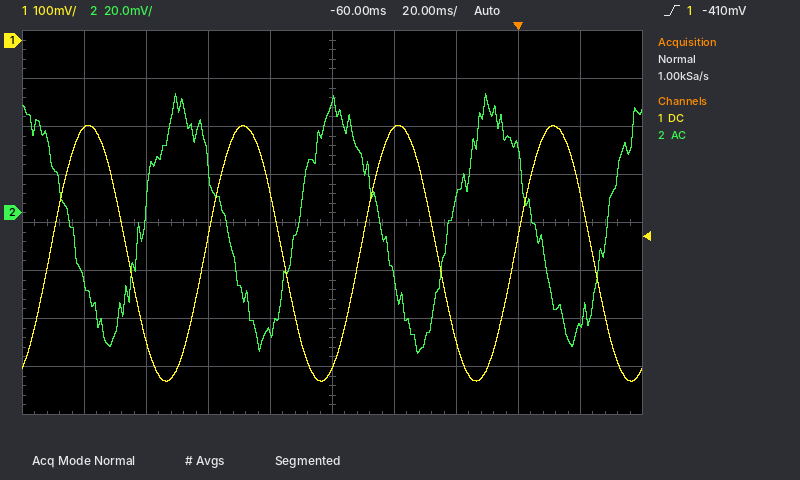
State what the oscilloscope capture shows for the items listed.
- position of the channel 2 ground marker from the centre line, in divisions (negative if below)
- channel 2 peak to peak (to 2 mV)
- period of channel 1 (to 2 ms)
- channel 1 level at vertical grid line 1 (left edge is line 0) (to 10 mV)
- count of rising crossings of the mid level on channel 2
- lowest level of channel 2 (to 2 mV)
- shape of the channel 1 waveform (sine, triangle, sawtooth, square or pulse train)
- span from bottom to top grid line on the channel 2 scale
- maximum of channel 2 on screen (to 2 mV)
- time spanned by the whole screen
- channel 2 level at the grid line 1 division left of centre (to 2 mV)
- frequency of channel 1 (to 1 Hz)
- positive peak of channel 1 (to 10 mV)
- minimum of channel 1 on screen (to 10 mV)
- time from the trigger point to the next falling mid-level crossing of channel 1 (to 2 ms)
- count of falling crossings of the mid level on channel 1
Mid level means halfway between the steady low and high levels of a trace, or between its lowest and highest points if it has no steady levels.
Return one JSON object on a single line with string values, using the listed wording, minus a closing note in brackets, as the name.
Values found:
{"position of the channel 2 ground marker from the centre line, in divisions": "+0.2 div", "channel 2 peak to peak": "108 mV", "period of channel 1": "50 ms", "channel 1 level at vertical grid line 1 (left edge is line 0)": "-180 mV", "count of rising crossings of the mid level on channel 2": "4", "lowest level of channel 2": "-58 mV", "shape of the channel 1 waveform": "sine", "span from bottom to top grid line on the channel 2 scale": "160 mV", "maximum of channel 2 on screen": "50 mV", "time spanned by the whole screen": "200 ms", "channel 2 level at the grid line 1 division left of centre": "-50 mV", "frequency of channel 1": "20 Hz", "positive peak of channel 1": "-180 mV", "minimum of channel 1 on screen": "-710 mV", "time from the trigger point to the next falling mid-level crossing of channel 1": "24 ms", "count of falling crossings of the mid level on channel 1": "4"}
